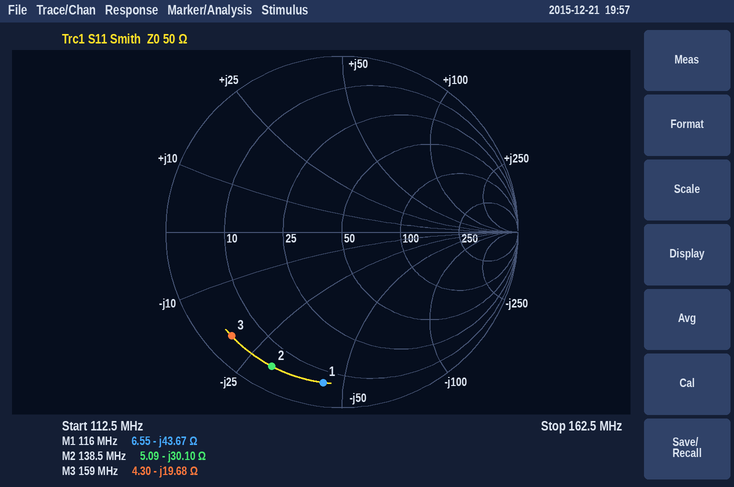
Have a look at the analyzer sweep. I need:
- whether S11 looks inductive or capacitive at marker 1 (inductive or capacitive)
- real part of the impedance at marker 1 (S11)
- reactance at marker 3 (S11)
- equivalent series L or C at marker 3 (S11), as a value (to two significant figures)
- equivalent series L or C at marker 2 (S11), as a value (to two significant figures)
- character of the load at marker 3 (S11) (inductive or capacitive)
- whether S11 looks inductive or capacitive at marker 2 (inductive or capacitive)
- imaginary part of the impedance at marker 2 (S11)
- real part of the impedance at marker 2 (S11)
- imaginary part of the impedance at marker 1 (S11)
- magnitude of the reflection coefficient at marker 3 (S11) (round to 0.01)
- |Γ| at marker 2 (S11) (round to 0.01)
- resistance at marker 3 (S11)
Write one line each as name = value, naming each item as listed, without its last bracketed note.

whether S11 looks inductive or capacitive at marker 1 = capacitive
real part of the impedance at marker 1 = 6.55 Ω
reactance at marker 3 = -19.68 Ω
equivalent series L or C at marker 3 (S11), as a value = 51 pF
equivalent series L or C at marker 2 (S11), as a value = 38 pF
character of the load at marker 3 (S11) = capacitive
whether S11 looks inductive or capacitive at marker 2 = capacitive
imaginary part of the impedance at marker 2 = -30.10 Ω
real part of the impedance at marker 2 = 5.09 Ω
imaginary part of the impedance at marker 1 = -43.67 Ω
magnitude of the reflection coefficient at marker 3 (S11) = 0.86
|Γ| at marker 2 (S11) = 0.86
resistance at marker 3 = 4.30 Ω
